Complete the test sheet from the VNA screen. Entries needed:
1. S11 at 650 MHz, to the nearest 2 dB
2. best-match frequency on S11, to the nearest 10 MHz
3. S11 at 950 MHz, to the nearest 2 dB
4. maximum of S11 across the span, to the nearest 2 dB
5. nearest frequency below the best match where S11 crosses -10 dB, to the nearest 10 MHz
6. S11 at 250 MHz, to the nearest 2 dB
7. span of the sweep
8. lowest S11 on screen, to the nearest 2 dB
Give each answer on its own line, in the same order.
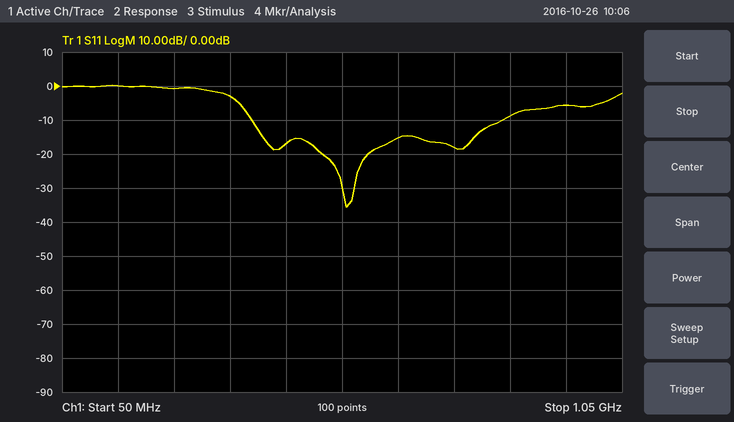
-16 dB
560 MHz
-6 dB
0 dB
390 MHz
0 dB
1 GHz
-36 dB
